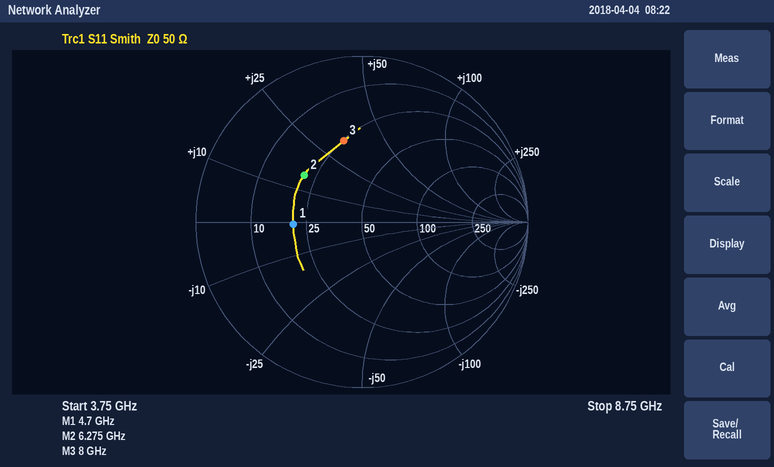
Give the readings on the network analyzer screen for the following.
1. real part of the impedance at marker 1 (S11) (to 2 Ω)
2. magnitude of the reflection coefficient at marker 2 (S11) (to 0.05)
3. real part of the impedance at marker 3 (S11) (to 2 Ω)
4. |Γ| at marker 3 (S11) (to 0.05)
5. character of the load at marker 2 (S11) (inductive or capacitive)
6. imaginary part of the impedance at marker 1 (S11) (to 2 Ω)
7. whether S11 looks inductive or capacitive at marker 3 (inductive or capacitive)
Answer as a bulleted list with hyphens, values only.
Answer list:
- 20 Ω
- 0.45
- 26 Ω
- 0.50
- inductive
- 0 Ω
- inductive
